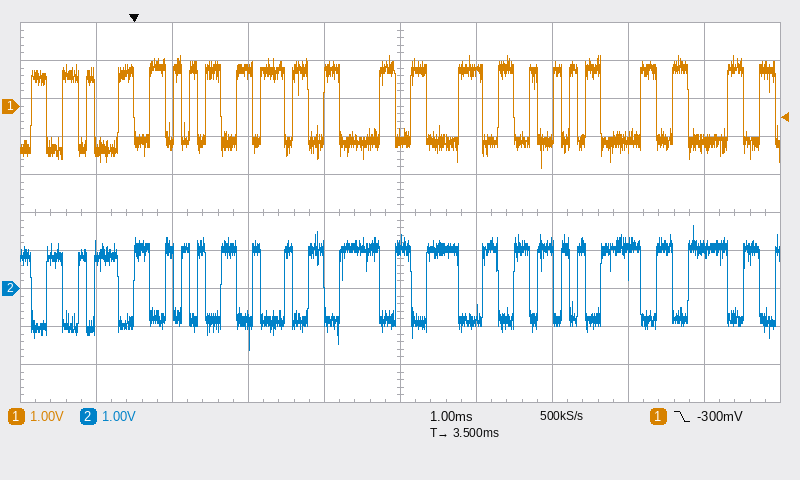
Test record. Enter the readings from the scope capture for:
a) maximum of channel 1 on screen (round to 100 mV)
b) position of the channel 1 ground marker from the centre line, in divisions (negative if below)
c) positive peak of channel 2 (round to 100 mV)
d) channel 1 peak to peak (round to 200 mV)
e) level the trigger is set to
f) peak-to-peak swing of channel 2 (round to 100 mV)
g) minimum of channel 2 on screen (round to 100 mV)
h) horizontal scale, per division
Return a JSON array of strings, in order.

["1.3 V", "+2.8 div", "1.7 V", "3.0 V", "-300 mV", "3.3 V", "-1.6 V", "1 ms"]
